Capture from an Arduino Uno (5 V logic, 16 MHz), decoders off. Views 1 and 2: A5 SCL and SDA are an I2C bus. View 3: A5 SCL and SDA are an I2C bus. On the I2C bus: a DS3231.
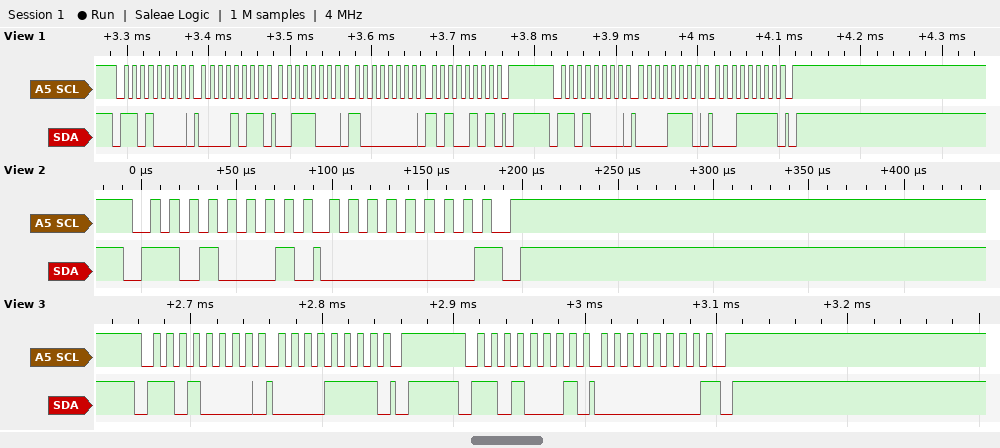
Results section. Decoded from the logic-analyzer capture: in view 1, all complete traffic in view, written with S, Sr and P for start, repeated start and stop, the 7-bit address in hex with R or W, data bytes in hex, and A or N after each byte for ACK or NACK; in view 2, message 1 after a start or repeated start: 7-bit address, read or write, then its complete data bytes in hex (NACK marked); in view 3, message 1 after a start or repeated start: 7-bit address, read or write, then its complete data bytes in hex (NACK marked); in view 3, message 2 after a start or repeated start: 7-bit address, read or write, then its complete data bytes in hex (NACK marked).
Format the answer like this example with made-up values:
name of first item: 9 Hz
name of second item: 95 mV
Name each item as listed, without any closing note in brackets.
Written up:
in view 1, all complete traffic in view, written with S, Sr and P for start, repeated start and stop, the 7-bit address in hex with R or W, data bytes in hex, and A or N after each byte for ACK or NACK: S 68W A 0B A 38 A 80 A A5 A P S 68W A 0E A 1F A P
in view 2, message 1 after a start or repeated start: 7-bit address, read or write, then its complete data bytes in hex: 0x68 read: 00 NACK
in view 3, message 1 after a start or repeated start: 7-bit address, read or write, then its complete data bytes in hex: 0x68 write: 0F
in view 3, message 2 after a start or repeated start: 7-bit address, read or write, then its complete data bytes in hex: 0x68 read: 00 NACK
